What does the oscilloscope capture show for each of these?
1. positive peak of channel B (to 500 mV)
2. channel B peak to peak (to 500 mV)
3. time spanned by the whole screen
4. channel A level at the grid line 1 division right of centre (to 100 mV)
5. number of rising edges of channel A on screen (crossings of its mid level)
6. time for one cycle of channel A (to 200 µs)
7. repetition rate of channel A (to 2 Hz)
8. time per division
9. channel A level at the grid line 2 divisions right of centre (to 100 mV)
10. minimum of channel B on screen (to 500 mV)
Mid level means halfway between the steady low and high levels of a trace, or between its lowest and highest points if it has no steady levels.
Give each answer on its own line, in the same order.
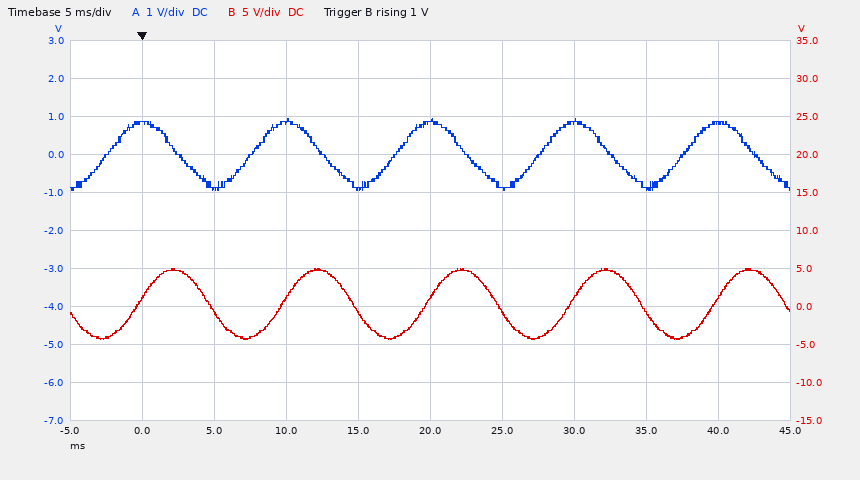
5.0 V
9.5 V
50 ms
-900 mV
5
10.0 ms
100 Hz
5 ms
900 mV
-4.5 V
